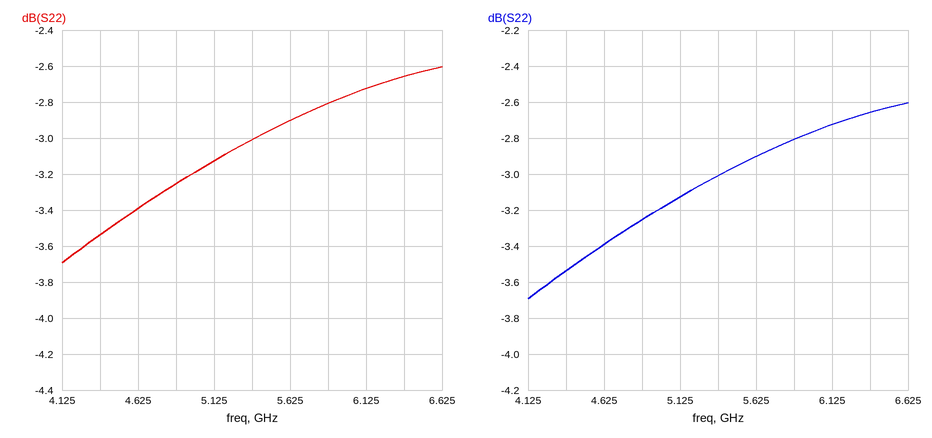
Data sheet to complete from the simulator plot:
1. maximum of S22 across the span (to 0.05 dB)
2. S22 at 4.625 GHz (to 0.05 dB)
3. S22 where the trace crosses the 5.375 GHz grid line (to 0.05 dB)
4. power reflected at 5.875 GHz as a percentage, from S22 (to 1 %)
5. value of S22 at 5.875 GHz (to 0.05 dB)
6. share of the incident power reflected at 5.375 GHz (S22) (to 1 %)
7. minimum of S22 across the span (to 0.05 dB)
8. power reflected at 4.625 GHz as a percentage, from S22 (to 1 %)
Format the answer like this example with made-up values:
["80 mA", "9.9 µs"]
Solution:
["-2.60 dB", "-3.40 dB", "-3.00 dB", "52 %", "-2.80 dB", "50 %", "-3.70 dB", "46 %"]
